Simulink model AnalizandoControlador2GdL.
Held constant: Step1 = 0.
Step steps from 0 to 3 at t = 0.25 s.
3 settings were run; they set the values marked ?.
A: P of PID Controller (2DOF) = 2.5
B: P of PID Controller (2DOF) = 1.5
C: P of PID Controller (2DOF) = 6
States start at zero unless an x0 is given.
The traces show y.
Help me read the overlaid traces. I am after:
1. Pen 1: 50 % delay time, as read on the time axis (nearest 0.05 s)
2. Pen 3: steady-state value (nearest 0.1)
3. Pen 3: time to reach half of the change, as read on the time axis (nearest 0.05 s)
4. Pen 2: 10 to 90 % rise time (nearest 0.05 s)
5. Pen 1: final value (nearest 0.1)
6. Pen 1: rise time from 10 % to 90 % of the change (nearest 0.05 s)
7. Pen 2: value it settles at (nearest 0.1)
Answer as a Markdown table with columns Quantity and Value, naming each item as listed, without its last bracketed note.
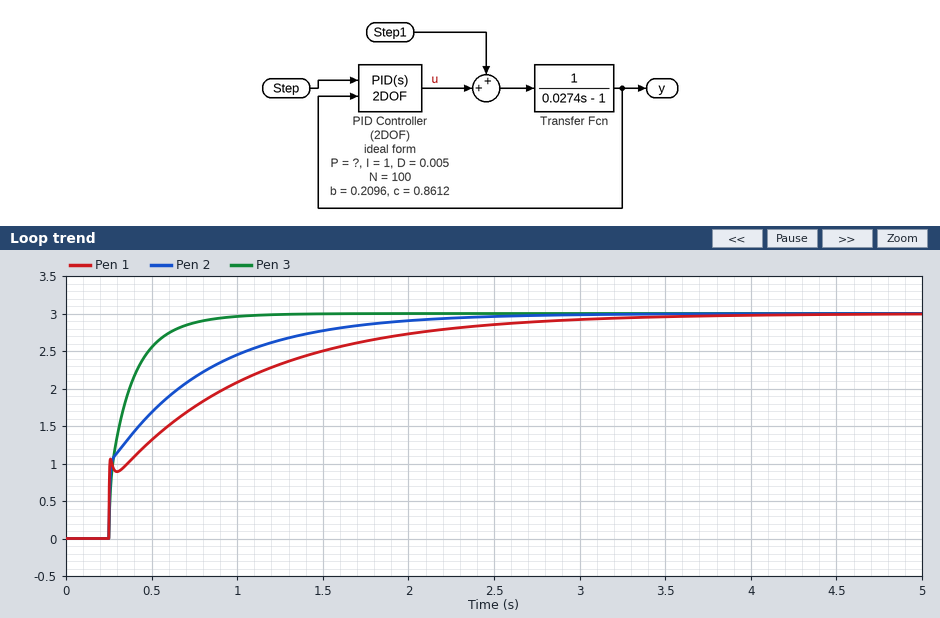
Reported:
| Quantity | Value |
|---|---|
| Pen 1: 50 % delay time, as read on the time axis | 0.60 s |
| Pen 3: steady-state value | 3.0 |
| Pen 3: time to reach half of the change, as read on the time axis | 0.30 s |
| Pen 2: 10 to 90 % rise time | 1.10 s |
| Pen 1: final value | 3.0 |
| Pen 1: rise time from 10 % to 90 % of the change | 1.65 s |
| Pen 2: value it settles at | 3.0 |
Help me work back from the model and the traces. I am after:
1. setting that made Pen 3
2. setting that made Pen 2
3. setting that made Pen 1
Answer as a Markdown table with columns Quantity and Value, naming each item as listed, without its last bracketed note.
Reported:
| Quantity | Value |
|---|---|
| setting that made Pen 3 | B |
| setting that made Pen 2 | A |
| setting that made Pen 1 | C |
